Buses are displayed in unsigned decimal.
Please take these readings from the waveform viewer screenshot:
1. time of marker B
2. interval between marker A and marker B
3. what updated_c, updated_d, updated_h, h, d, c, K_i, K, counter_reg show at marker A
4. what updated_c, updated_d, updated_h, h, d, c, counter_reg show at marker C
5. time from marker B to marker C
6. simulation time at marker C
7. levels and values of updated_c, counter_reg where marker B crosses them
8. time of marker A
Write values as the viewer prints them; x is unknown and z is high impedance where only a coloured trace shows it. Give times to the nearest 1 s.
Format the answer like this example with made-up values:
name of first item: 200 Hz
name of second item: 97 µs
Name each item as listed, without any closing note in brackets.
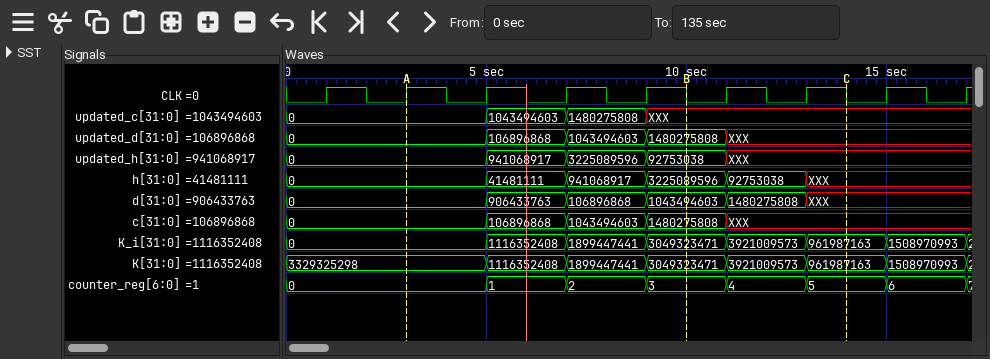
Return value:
time of marker B: 10 s
interval between marker A and marker B: 7 s
what updated_c, updated_d, updated_h, h, d, c, K_i, K, counter_reg show at marker A: updated_c=0, updated_d=0, updated_h=0, h=0, d=0, c=0, K_i=0, K=3329325298, counter_reg=0
what updated_c, updated_d, updated_h, h, d, c, counter_reg show at marker C: updated_c=XXX, updated_d=XXX, updated_h=XXX, h=XXX, d=XXX, c=XXX, counter_reg=5
time from marker B to marker C: 4 s
simulation time at marker C: 14 s
levels and values of updated_c, counter_reg where marker B crosses them: updated_c=XXX, counter_reg=3
time of marker A: 3 s
